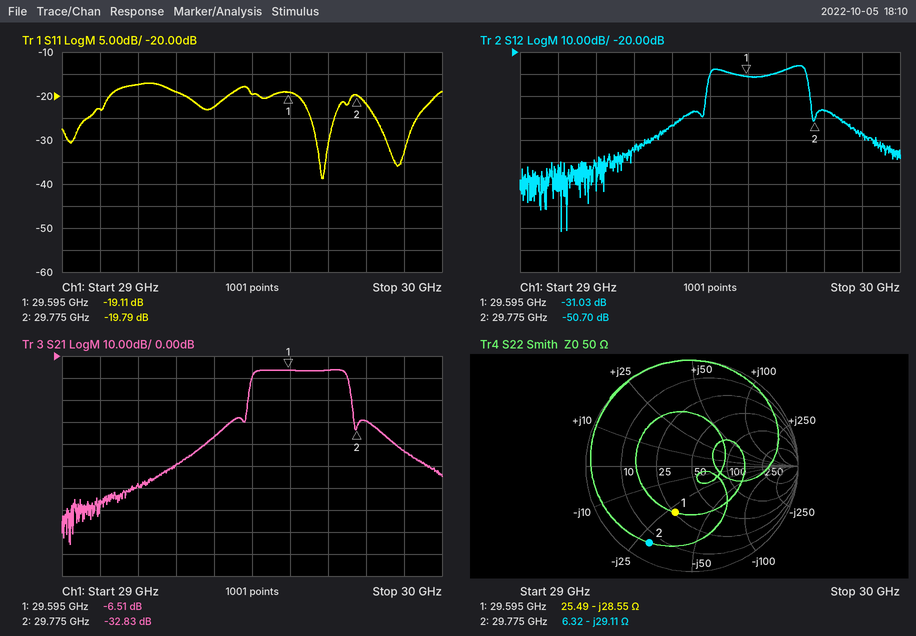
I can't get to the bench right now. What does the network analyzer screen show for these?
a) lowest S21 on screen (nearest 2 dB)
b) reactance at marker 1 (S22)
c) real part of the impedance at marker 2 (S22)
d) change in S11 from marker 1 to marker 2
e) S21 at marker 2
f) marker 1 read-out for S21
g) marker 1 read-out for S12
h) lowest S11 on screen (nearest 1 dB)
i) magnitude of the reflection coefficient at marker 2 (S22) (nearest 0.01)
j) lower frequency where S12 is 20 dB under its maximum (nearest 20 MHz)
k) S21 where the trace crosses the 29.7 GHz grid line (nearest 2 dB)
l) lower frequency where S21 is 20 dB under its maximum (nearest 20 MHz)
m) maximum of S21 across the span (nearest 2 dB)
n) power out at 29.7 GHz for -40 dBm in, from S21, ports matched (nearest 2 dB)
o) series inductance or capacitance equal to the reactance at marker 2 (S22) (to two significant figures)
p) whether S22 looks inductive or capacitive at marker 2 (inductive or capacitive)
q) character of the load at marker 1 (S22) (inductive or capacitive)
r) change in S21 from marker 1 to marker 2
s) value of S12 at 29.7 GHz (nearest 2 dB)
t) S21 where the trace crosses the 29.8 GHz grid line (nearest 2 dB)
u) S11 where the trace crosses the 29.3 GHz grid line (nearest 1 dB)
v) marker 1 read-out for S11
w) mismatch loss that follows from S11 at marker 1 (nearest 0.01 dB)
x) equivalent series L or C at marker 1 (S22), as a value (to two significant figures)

-86 dB
-28.55 Ω
6.32 Ω
-0.68 dB
-32.83 dB
-6.51 dB
-31.03 dB
-39 dB
0.83
29.48 GHz
-6 dB
29.48 GHz
-6 dB
-46 dBm
180 fF
capacitive
capacitive
-26.32 dB
-28 dB
-30 dB
-19 dB
-19.11 dB
0.05 dB
190 fF
